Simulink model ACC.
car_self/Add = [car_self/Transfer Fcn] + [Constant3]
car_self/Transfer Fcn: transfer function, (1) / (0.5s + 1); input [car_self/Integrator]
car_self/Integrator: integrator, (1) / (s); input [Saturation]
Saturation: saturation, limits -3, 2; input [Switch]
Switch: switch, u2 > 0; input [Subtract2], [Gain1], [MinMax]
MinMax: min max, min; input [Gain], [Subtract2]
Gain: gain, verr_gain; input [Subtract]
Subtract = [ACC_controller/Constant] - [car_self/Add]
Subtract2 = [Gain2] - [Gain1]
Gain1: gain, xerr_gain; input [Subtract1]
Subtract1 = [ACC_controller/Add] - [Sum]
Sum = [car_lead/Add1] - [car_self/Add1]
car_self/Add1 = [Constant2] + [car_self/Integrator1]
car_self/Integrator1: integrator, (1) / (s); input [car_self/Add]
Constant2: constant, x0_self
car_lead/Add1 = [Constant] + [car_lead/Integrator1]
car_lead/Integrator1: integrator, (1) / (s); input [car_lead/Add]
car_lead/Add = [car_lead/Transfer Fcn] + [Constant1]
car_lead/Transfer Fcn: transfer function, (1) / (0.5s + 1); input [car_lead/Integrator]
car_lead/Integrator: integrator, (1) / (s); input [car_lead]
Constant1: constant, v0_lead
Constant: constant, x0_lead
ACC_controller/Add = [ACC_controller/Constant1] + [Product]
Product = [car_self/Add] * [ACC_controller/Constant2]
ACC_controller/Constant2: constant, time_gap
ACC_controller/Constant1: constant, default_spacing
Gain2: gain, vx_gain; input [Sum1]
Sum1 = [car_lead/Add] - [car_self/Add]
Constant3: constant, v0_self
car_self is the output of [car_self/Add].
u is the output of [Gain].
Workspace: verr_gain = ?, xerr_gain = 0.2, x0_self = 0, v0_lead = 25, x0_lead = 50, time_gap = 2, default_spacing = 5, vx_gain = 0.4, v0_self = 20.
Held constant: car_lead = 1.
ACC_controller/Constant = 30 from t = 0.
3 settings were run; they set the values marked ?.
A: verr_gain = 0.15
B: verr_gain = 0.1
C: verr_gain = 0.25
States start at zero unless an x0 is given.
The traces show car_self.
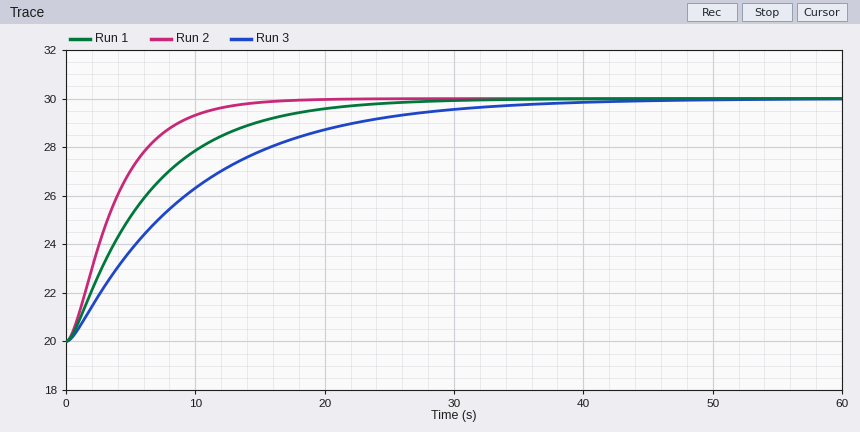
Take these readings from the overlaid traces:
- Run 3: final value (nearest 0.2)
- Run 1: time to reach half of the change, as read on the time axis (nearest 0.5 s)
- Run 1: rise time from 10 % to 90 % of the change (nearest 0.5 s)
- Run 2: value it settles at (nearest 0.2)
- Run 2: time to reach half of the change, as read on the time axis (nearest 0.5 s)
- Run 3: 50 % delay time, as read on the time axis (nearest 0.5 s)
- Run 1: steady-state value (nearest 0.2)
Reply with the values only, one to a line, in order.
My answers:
30.0
5.0 s
13.5 s
30.0
3.0 s
7.0 s
30.0
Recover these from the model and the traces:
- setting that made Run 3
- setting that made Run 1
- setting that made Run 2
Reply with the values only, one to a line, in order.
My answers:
B
A
C
